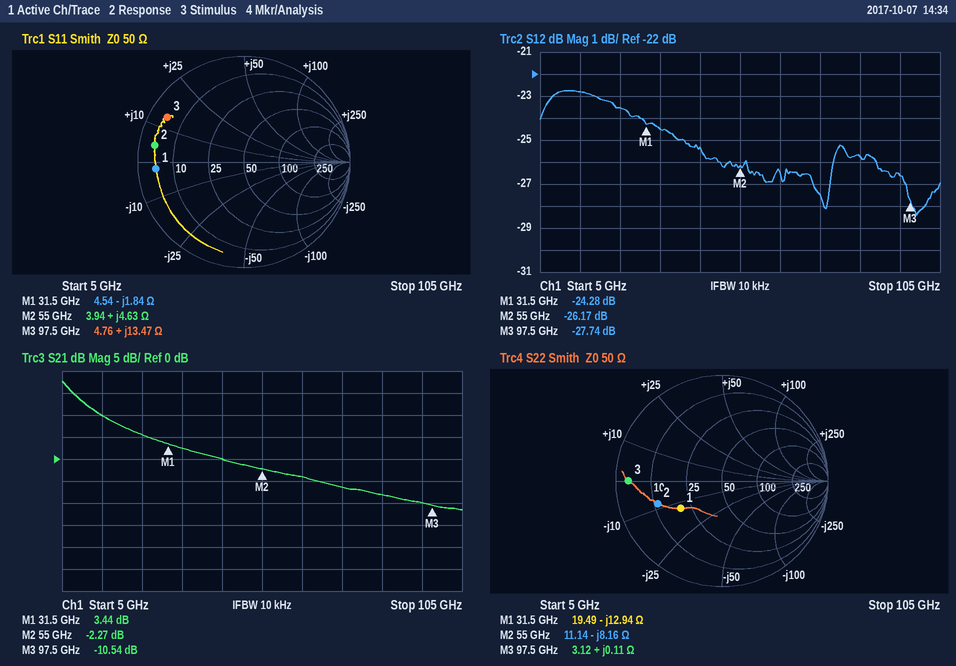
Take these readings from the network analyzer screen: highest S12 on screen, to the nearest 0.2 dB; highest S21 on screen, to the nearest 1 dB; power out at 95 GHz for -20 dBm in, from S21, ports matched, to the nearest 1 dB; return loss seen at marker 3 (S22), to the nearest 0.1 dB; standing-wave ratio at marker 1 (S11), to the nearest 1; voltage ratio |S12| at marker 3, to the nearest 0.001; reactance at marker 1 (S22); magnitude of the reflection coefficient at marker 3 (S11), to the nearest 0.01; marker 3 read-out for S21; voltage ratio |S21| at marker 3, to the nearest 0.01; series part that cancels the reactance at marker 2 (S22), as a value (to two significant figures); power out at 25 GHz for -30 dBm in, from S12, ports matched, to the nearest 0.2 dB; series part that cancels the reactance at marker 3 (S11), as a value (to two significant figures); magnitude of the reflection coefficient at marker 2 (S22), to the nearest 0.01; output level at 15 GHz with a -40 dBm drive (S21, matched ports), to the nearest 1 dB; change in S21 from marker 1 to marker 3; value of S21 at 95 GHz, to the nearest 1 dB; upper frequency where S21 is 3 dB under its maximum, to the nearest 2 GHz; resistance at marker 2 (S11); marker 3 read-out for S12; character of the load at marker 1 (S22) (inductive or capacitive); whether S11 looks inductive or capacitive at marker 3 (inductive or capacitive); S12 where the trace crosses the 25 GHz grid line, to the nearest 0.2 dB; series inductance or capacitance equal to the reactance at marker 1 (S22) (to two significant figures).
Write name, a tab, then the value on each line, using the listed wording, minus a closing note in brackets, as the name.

highest S12 on screen, to the nearest 0.2 dB	-22.8 dB
highest S21 on screen, to the nearest 1 dB	18 dB
power out at 95 GHz for -20 dBm in, from S21, ports matched, to the nearest 1 dB	-30 dBm
return loss seen at marker 3 (S22), to the nearest 0.1 dB	1.1 dB
standing-wave ratio at marker 1 (S11), to the nearest 1	11
voltage ratio |S12| at marker 3, to the nearest 0.001	0.041
reactance at marker 1	-12.94 Ω
magnitude of the reflection coefficient at marker 3 (S11), to the nearest 0.01	0.84
marker 3 read-out for S21	-10.54 dB
voltage ratio |S21| at marker 3, to the nearest 0.01	0.30
series part that cancels the reactance at marker 2 (S22), as a value	24 pH
power out at 25 GHz for -30 dBm in, from S12, ports matched, to the nearest 0.2 dB	-53.6 dBm
series part that cancels the reactance at marker 3 (S11), as a value	120 fF
magnitude of the reflection coefficient at marker 2 (S22), to the nearest 0.01	0.64
output level at 15 GHz with a -40 dBm drive (S21, matched ports), to the nearest 1 dB	-30 dBm
change in S21 from marker 1 to marker 3	-13.98 dB
value of S21 at 95 GHz, to the nearest 1 dB	-10 dB
upper frequency where S21 is 3 dB under its maximum, to the nearest 2 GHz	8 GHz
resistance at marker 2	3.94 Ω
marker 3 read-out for S12	-27.74 dB
character of the load at marker 1 (S22)	capacitive
whether S11 looks inductive or capacitive at marker 3	inductive
S12 where the trace crosses the 25 GHz grid line, to the nearest 0.2 dB	-23.6 dB
series inductance or capacitance equal to the reactance at marker 1 (S22)	390 fF
